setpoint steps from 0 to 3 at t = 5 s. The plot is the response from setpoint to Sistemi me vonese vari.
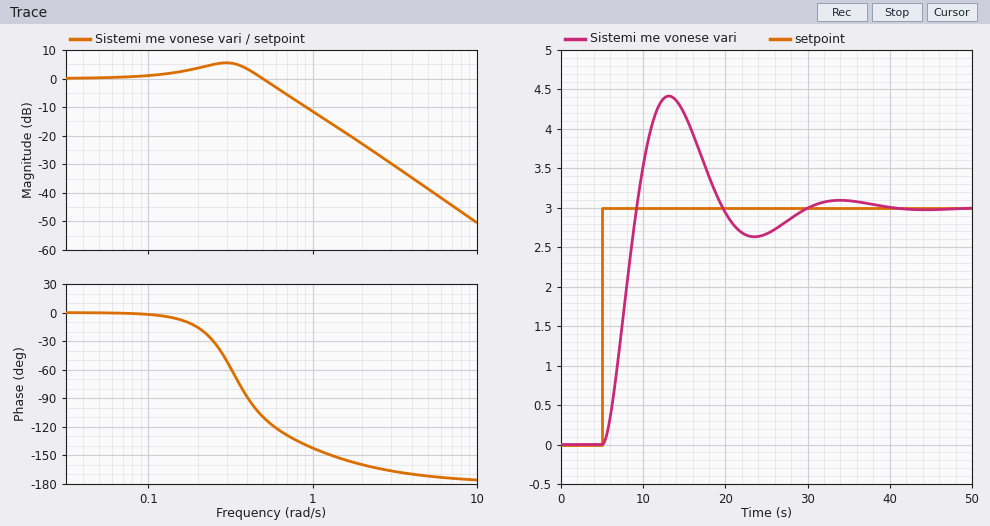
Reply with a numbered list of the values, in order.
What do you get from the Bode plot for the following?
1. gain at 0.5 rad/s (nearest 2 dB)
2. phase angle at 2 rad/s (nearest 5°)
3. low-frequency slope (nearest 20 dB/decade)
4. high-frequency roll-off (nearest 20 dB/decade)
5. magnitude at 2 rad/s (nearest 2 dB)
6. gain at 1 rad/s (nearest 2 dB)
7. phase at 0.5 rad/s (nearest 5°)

1. 0 dB
2. -160°
3. 0 dB/decade
4. -40 dB/decade
5. -22 dB
6. -12 dB
7. -110°
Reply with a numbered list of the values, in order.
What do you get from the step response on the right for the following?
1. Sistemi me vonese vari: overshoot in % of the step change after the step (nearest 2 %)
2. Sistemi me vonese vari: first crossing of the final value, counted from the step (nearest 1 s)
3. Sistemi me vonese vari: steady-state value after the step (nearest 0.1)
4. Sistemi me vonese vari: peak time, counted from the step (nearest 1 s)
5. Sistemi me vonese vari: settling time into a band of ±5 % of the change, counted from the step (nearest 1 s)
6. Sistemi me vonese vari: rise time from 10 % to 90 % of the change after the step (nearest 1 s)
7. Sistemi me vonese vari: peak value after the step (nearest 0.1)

1. 48 %
2. 4 s
3. 3.0
4. 8 s
5. 23 s
6. 3 s
7. 4.4
